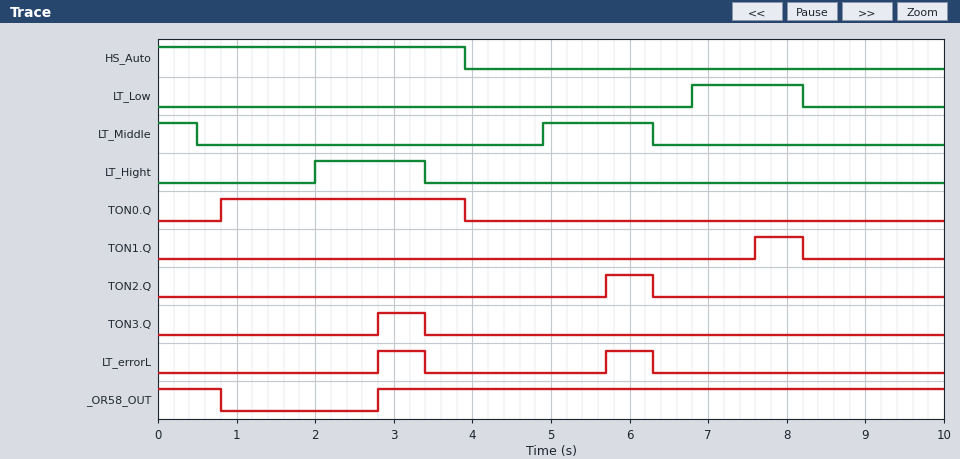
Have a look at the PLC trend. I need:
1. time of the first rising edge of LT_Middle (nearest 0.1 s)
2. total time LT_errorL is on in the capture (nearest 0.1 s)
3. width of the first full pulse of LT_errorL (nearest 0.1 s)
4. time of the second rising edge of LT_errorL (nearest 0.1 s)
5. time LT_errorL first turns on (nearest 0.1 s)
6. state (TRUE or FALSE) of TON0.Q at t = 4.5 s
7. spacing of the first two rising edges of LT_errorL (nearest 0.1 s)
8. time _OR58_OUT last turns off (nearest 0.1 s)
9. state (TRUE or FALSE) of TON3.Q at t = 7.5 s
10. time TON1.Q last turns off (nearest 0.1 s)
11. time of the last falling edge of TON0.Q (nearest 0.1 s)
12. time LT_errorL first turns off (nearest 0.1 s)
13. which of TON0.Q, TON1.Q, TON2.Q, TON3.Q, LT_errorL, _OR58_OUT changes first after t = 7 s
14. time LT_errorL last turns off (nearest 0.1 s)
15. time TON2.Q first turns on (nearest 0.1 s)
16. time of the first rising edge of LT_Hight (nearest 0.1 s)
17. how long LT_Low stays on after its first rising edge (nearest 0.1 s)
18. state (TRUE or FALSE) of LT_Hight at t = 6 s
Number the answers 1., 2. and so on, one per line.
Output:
1. 4.9 s
2. 1.2 s
3. 0.6 s
4. 5.7 s
5. 2.8 s
6. FALSE
7. 2.9 s
8. 0.8 s
9. FALSE
10. 8.2 s
11. 3.9 s
12. 3.4 s
13. TON1.Q
14. 6.3 s
15. 5.7 s
16. 2.0 s
17. 1.4 s
18. FALSE
